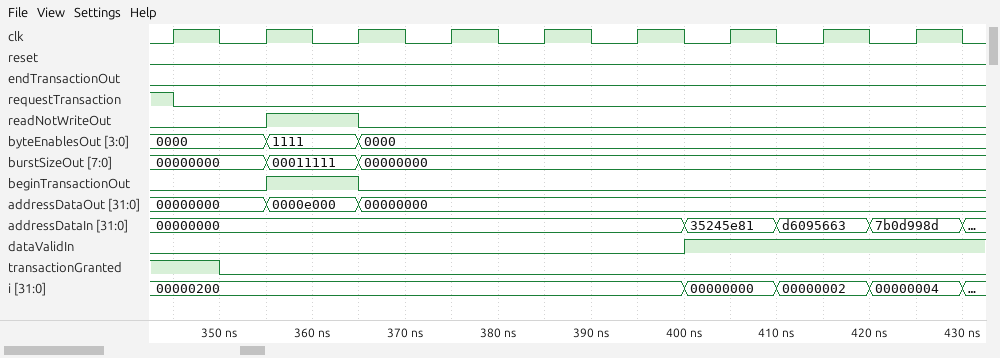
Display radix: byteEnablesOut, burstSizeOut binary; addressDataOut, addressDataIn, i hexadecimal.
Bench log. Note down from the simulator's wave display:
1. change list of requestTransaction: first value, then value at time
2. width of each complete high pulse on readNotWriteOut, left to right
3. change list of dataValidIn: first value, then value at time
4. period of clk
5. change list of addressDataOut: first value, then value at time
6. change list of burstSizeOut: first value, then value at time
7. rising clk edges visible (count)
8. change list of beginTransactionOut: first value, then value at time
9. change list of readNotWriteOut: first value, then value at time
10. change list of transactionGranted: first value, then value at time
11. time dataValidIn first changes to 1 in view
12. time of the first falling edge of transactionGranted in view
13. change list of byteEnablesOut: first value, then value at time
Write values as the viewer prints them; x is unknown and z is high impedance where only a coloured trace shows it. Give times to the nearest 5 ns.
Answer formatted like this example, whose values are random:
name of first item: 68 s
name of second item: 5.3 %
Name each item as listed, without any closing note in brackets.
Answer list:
change list of requestTransaction: first value, then value at time: 1, 0 at 345 ns
width of each complete high pulse on readNotWriteOut, left to right: 10 ns
change list of dataValidIn: first value, then value at time: 0, 1 at 400 ns
period of clk: 10 ns
change list of addressDataOut: first value, then value at time: 00000000, 0000e000 at 355 ns, 00000000 at 365 ns
change list of burstSizeOut: first value, then value at time: 00000000, 00011111 at 355 ns, 00000000 at 365 ns
rising clk edges visible: 9
change list of beginTransactionOut: first value, then value at time: 0, 1 at 355 ns, 0 at 365 ns
change list of readNotWriteOut: first value, then value at time: 0, 1 at 355 ns, 0 at 365 ns
change list of transactionGranted: first value, then value at time: 1, 0 at 350 ns
time dataValidIn first changes to 1 in view: 400 ns
time of the first falling edge of transactionGranted in view: 350 ns
change list of byteEnablesOut: first value, then value at time: 0000, 1111 at 355 ns, 0000 at 365 ns
